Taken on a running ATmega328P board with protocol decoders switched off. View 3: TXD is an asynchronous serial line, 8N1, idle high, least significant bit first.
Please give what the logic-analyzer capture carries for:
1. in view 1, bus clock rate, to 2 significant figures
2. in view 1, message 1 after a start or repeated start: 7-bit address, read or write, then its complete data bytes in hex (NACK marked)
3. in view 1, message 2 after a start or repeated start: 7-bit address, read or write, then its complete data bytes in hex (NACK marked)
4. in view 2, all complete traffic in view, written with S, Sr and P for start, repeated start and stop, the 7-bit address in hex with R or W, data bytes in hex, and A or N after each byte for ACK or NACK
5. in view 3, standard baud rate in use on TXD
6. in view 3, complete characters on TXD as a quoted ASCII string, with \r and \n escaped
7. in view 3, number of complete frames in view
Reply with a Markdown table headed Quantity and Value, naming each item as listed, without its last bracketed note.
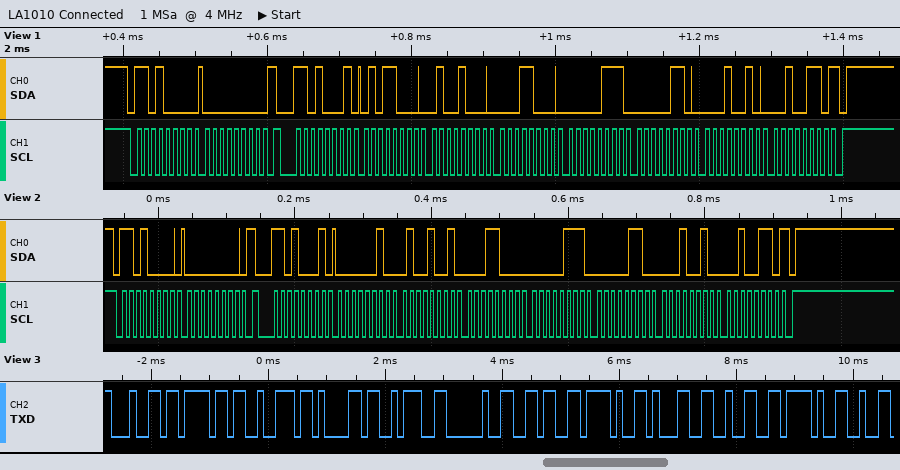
| Quantity | Value |
|---|---|
| in view 1, bus clock rate, to 2 significant figures | 100 kHz |
| in view 1, message 1 after a start or repeated start: 7-bit address, read or write, then its complete data bytes in hex | 0x68 write: 00 |
| in view 1, message 2 after a start or repeated start: 7-bit address, read or write, then its complete data bytes in hex | 0x68 read: 58 48 18 07 06 12 26 NACK |
| in view 2, all complete traffic in view, written with S, Sr and P for start, repeated start and stop, the 7-bit address in hex with R or W, data bytes in hex, and A or N after each byte for ACK or NACK | S 68W A 00 A Sr 68R A 02 A 49 A 18 A 07 A 06 A 12 A 26 N P |
| in view 3, standard baud rate in use on TXD | 9600 baud |
| in view 3, complete characters on TXD as a quoted ASCII string, with \r and \n escaped | "dora: 6/12/" |
| in view 3, number of complete frames in view | 11 |
